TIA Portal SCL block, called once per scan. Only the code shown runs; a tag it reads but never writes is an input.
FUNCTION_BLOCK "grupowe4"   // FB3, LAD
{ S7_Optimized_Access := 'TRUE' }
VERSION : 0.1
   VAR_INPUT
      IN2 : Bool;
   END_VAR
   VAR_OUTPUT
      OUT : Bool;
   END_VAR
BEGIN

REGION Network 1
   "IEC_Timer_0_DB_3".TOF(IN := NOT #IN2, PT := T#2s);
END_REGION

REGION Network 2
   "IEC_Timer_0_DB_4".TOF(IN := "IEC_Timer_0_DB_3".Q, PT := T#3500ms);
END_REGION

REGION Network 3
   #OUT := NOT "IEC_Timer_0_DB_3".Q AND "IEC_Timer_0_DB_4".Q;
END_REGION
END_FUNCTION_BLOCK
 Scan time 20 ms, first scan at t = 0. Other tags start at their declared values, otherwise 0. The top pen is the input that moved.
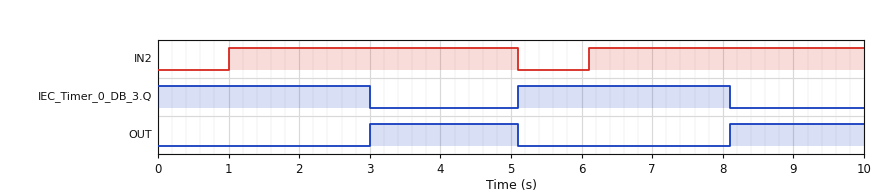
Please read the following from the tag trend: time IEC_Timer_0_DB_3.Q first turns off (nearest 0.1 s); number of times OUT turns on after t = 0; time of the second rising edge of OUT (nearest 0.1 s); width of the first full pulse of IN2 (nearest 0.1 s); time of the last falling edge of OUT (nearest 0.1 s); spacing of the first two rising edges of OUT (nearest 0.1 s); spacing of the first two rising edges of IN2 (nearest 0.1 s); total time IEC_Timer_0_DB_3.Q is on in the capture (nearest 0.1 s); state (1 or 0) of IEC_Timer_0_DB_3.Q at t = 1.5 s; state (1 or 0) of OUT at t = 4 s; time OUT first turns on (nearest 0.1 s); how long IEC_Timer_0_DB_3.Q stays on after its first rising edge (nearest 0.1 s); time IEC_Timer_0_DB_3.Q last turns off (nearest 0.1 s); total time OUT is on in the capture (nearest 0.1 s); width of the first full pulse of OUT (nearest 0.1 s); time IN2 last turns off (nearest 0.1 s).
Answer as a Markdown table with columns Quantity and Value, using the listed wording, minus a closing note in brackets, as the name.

| Quantity | Value |
|---|---|
| time IEC_Timer_0_DB_3.Q first turns off | 3.0 s |
| number of times OUT turns on after t = 0 | 2 |
| time of the second rising edge of OUT | 8.1 s |
| width of the first full pulse of IN2 | 4.1 s |
| time of the last falling edge of OUT | 5.1 s |
| spacing of the first two rising edges of OUT | 5.1 s |
| spacing of the first two rising edges of IN2 | 5.1 s |
| total time IEC_Timer_0_DB_3.Q is on in the capture | 6.0 s |
| state (1 or 0) of IEC_Timer_0_DB_3.Q at t = 1.5 s | 1 |
| state (1 or 0) of OUT at t = 4 s | 1 |
| time OUT first turns on | 3.0 s |
| how long IEC_Timer_0_DB_3.Q stays on after its first rising edge | 3.0 s |
| time IEC_Timer_0_DB_3.Q last turns off | 8.1 s |
| total time OUT is on in the capture | 4.0 s |
| width of the first full pulse of OUT | 2.1 s |
| time IN2 last turns off | 5.1 s |
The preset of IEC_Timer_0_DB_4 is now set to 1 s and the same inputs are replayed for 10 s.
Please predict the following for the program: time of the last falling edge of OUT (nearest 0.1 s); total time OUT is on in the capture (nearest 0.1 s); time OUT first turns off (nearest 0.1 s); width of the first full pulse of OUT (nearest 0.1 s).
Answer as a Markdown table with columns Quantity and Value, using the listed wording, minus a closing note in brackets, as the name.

| Quantity | Value |
|---|---|
| time of the last falling edge of OUT | 9.1 s |
| total time OUT is on in the capture | 2.0 s |
| time OUT first turns off | 4.0 s |
| width of the first full pulse of OUT | 1.0 s |
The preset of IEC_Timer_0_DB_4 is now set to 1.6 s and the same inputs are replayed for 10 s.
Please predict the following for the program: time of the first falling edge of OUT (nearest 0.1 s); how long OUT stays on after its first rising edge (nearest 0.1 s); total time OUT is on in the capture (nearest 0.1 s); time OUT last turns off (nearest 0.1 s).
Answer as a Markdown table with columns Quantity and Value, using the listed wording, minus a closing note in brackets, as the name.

| Quantity | Value |
|---|---|
| time of the first falling edge of OUT | 4.6 s |
| how long OUT stays on after its first rising edge | 1.6 s |
| total time OUT is on in the capture | 3.2 s |
| time OUT last turns off | 9.7 s |
